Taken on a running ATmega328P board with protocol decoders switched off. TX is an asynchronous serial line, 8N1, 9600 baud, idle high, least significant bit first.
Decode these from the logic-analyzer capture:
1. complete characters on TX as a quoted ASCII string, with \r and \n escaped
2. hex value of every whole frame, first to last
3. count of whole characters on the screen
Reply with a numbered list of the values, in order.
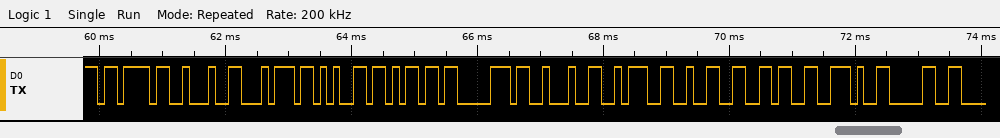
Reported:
1. "{\"temp\":26.0"
2. 7B 22 74 65 6D 70 22 3A 32 36 2E 30
3. 12
